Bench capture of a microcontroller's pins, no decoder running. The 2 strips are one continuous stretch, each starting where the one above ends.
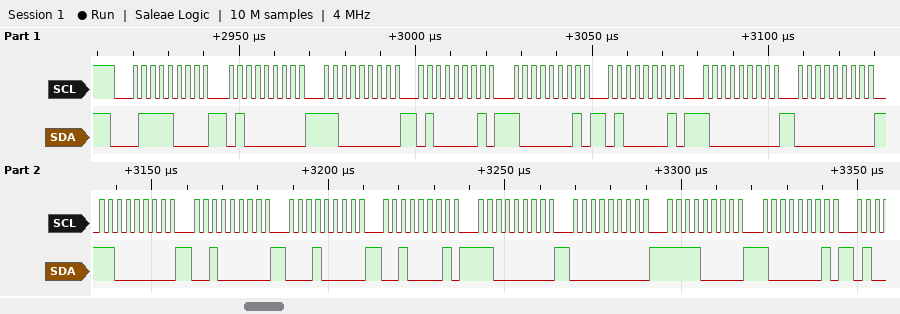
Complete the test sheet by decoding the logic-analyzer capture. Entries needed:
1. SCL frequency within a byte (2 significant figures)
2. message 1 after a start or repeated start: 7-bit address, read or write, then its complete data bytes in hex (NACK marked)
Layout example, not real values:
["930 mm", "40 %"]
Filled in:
["400 kHz", "0x3C write: 40 C0 41 81 41 80 00 C0 20 10 21 C0 00 F0 81"]
